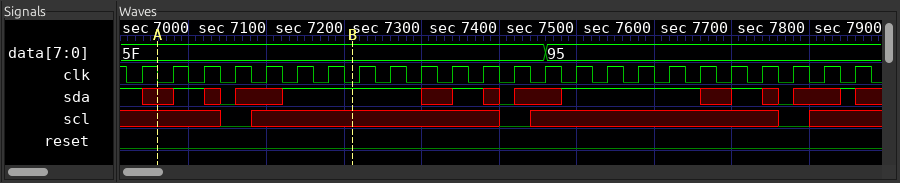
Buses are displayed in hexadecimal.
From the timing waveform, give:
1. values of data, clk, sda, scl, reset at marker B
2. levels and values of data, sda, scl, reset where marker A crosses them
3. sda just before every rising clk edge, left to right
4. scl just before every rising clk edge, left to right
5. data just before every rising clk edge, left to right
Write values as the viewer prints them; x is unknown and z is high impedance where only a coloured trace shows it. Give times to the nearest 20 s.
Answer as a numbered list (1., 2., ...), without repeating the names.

1. data=5F, clk=0, sda=1, scl=x, reset=0
2. data=5F, sda=x, scl=x, reset=0
3. 1 x 1 0 x 1 1 1 1 1 x 1 0 x 1 1 1 1 1 x 1 0 x 1
4. x x x 0 x x x x x x x x 0 x x x x x x x x 0 x x
5. 5F, 5F, 5F, 5F, 5F, 5F, 5F, 5F, 5F, 5F, 5F, 5F, 5F, 5F, 95, 95, 95, 95, 95, 95, 95, 95, 95, 95
